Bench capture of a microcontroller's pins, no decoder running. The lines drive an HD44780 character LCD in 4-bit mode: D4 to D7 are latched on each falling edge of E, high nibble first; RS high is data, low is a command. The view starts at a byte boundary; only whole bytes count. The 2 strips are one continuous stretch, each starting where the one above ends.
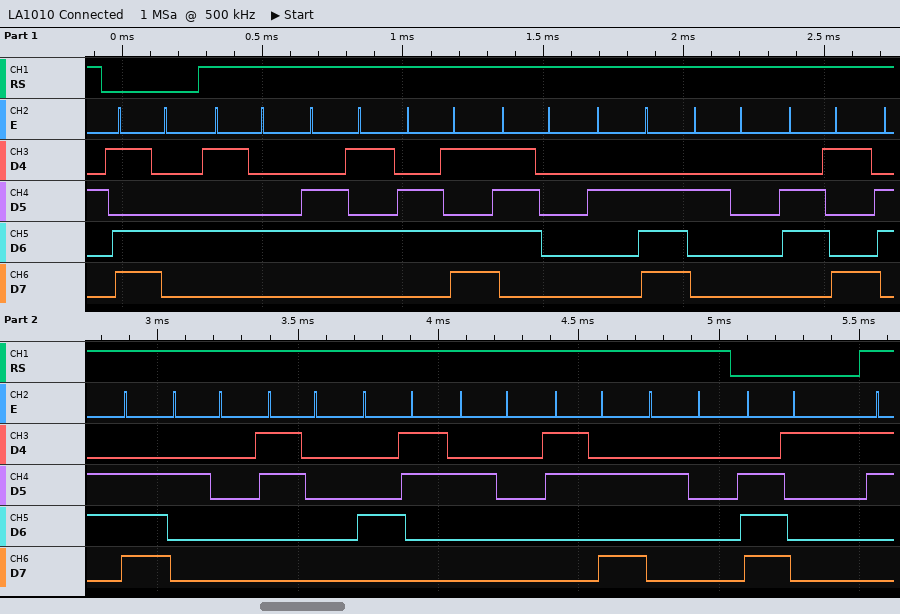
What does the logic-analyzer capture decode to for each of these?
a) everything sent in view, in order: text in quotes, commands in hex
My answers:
0xD4 "Temp. in 0C : " 0xE1
